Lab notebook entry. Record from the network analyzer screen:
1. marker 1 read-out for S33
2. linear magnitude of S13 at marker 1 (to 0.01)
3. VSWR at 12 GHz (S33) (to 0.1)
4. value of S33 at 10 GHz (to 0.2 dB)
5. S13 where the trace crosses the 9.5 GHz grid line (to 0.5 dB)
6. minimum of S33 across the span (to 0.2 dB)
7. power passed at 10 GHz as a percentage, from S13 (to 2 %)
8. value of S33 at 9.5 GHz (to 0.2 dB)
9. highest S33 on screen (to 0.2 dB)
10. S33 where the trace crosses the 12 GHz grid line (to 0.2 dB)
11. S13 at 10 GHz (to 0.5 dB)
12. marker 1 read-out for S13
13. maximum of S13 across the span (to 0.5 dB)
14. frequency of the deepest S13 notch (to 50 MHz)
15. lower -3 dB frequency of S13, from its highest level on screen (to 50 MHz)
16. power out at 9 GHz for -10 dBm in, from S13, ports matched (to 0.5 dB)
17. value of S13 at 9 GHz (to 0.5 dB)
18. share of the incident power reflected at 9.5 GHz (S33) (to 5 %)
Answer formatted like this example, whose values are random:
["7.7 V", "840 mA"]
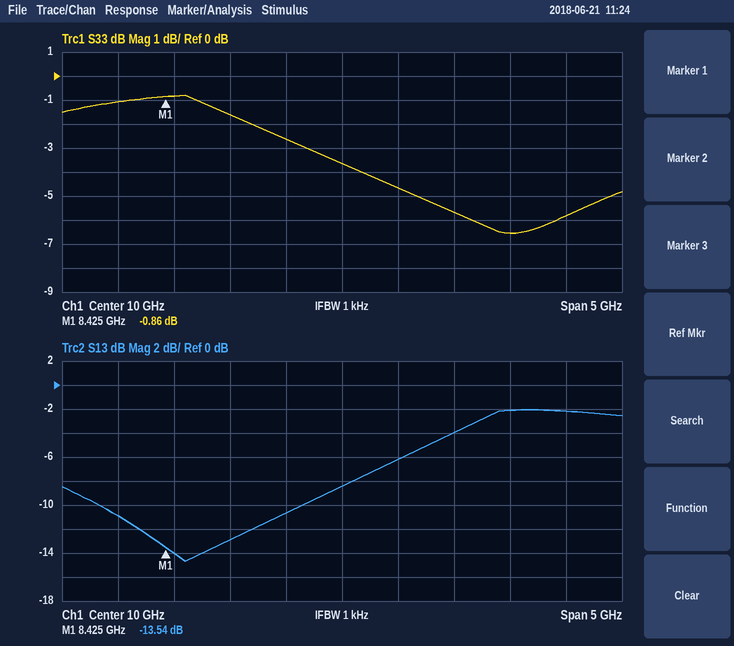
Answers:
["-0.86 dB", "0.21", "3.1", "-3.6 dB", "-10.5 dB", "-6.6 dB", "14 %", "-2.6 dB", "-0.8 dB", "-5.8 dB", "-8.5 dB", "-13.54 dB", "-2.0 dB", "8.60 GHz", "10.75 GHz", "-23.0 dBm", "-13.0 dB", "55 %"]
